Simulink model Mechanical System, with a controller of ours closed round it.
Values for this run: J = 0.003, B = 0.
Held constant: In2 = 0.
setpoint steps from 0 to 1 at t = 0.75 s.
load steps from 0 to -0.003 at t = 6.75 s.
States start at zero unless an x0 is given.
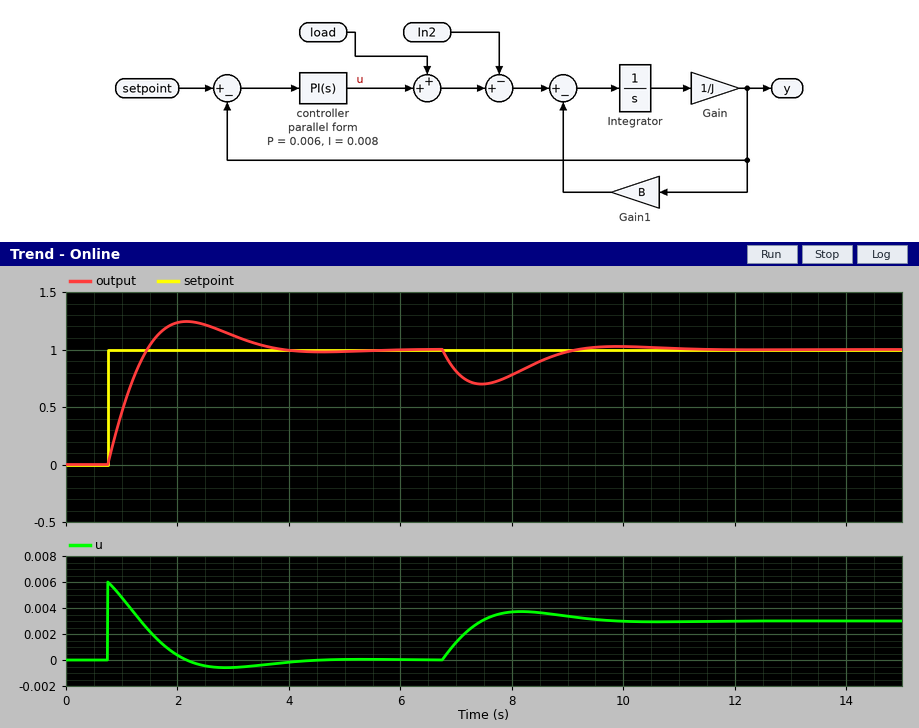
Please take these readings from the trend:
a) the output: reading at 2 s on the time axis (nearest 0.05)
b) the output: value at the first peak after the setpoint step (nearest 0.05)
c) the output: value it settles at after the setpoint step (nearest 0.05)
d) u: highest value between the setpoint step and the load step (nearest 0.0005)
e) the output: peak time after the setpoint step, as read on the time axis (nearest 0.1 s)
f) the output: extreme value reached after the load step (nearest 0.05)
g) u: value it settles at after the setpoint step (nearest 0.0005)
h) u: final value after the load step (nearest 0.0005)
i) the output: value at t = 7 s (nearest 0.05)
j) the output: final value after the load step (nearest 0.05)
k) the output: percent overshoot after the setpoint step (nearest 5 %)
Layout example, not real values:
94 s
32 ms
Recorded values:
1.25
1.25
1.00
0.0060
2.2 s
0.70
0.0000
0.0030
0.80
1.00
25 %
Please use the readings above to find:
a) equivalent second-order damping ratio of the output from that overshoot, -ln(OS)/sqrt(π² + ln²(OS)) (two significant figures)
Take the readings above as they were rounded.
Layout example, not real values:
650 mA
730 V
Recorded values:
0.40
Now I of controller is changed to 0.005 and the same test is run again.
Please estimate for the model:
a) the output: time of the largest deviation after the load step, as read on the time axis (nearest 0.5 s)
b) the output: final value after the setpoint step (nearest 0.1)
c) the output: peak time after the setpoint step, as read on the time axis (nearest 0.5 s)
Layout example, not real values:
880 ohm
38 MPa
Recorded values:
7.5 s
1.0
2.5 s
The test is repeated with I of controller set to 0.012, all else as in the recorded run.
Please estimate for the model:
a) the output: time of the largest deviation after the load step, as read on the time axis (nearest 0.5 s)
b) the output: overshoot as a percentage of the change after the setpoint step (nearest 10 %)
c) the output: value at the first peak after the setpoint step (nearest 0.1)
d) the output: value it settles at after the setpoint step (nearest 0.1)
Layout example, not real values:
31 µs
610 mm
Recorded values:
7.5 s
30 %
1.3
1.0
